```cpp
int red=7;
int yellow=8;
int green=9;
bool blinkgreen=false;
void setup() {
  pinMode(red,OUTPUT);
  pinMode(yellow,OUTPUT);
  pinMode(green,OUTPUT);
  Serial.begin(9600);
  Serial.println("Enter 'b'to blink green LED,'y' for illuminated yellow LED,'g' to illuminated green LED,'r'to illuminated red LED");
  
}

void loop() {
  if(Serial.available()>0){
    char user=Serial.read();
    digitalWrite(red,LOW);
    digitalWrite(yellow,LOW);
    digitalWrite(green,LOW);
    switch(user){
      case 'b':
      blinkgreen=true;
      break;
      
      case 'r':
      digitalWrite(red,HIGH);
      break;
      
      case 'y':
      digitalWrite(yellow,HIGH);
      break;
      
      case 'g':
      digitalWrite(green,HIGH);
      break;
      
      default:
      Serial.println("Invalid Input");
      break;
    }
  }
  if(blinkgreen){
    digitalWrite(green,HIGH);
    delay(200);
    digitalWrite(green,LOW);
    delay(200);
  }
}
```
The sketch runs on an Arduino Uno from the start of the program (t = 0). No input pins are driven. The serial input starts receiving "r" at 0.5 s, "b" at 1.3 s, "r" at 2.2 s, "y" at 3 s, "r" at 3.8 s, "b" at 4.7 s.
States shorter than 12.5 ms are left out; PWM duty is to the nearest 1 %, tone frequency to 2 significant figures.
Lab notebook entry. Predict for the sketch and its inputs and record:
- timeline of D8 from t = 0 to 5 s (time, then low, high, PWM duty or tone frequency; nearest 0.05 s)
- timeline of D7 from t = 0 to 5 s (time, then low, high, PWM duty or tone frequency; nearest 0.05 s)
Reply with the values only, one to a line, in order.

0 s low; 3.3 s high; 4.1 s low
0 s low; 0.5 s high; 1.3 s low; 2.5 s high; 3.3 s low; 4.1 s high; 4.9 s low
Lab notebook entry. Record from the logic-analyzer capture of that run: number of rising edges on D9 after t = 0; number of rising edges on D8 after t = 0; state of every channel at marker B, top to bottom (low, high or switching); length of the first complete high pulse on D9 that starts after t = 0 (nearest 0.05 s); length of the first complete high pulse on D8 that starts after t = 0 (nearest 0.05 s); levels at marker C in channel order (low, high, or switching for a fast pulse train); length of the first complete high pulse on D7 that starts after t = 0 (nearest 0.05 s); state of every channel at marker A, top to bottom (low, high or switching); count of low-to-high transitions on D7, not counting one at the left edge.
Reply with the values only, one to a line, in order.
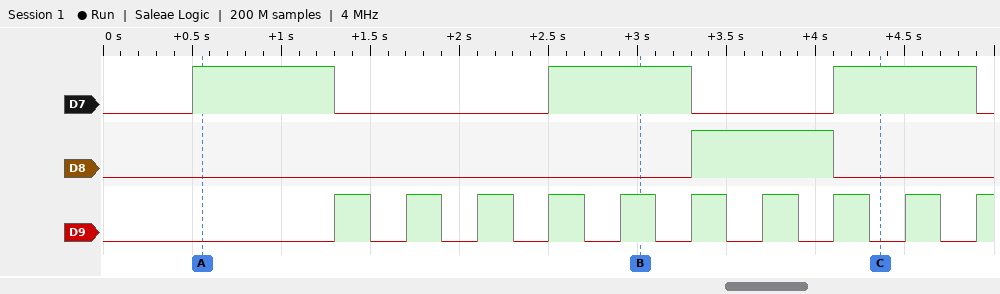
10
1
D7 high, D8 low, D9 high
0.20 s
0.80 s
D7 high, D8 low, D9 low
0.80 s
D7 high, D8 low, D9 low
3
